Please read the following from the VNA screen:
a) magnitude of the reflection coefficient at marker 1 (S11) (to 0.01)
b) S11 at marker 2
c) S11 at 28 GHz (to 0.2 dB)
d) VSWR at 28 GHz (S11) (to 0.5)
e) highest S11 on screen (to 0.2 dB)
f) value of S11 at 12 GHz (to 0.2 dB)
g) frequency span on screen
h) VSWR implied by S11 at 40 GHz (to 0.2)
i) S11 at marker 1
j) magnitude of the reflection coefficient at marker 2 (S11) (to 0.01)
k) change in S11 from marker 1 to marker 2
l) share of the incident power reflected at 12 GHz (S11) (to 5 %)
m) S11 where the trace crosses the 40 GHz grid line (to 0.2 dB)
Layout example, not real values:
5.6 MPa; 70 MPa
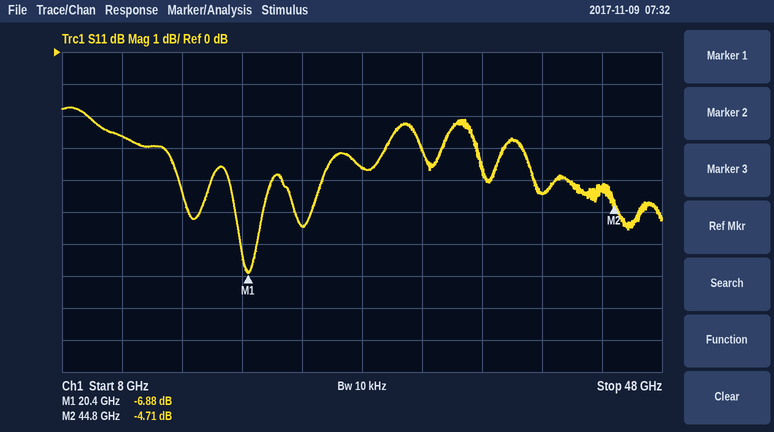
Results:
0.45; -4.71 dB; -3.6 dB; 5.0; -1.8 dB; -2.6 dB; 40 GHz; 4.0; -6.88 dB; 0.58; 2.17 dB; 55 %; -4.4 dB
